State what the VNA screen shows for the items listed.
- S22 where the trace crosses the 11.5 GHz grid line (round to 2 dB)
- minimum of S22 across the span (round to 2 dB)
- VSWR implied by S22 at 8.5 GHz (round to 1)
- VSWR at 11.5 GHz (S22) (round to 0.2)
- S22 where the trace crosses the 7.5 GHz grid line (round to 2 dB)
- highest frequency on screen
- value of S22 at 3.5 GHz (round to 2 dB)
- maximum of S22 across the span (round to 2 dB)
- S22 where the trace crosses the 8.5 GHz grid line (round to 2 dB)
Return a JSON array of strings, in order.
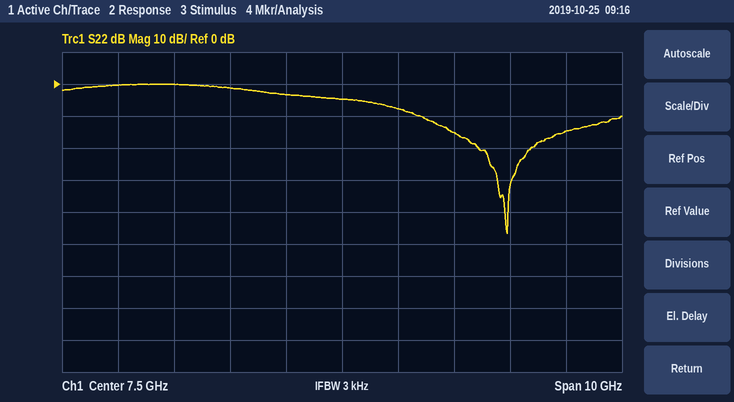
["-14 dB", "-46 dB", "2", "1.4", "-4 dB", "12.5 GHz", "0 dB", "0 dB", "-8 dB"]
